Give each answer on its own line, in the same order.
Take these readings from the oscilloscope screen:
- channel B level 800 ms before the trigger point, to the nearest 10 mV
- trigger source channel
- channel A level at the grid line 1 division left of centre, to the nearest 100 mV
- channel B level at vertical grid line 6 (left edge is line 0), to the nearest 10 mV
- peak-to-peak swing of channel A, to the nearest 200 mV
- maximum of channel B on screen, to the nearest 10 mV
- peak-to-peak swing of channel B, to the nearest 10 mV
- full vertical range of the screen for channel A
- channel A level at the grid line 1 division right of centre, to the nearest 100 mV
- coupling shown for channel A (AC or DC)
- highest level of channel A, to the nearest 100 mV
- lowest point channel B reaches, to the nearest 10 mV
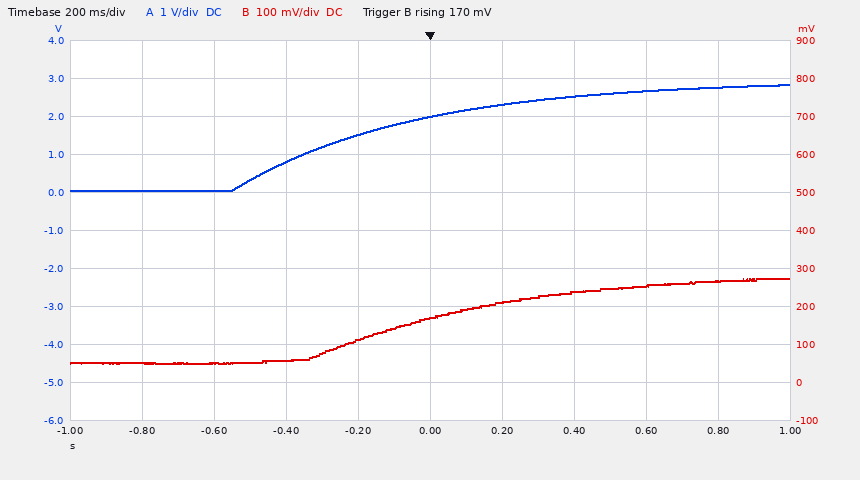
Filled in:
50 mV
channel B
1.5 V
210 mV
2.8 V
270 mV
220 mV
10 V
2.3 V
DC
2.8 V
50 mV
